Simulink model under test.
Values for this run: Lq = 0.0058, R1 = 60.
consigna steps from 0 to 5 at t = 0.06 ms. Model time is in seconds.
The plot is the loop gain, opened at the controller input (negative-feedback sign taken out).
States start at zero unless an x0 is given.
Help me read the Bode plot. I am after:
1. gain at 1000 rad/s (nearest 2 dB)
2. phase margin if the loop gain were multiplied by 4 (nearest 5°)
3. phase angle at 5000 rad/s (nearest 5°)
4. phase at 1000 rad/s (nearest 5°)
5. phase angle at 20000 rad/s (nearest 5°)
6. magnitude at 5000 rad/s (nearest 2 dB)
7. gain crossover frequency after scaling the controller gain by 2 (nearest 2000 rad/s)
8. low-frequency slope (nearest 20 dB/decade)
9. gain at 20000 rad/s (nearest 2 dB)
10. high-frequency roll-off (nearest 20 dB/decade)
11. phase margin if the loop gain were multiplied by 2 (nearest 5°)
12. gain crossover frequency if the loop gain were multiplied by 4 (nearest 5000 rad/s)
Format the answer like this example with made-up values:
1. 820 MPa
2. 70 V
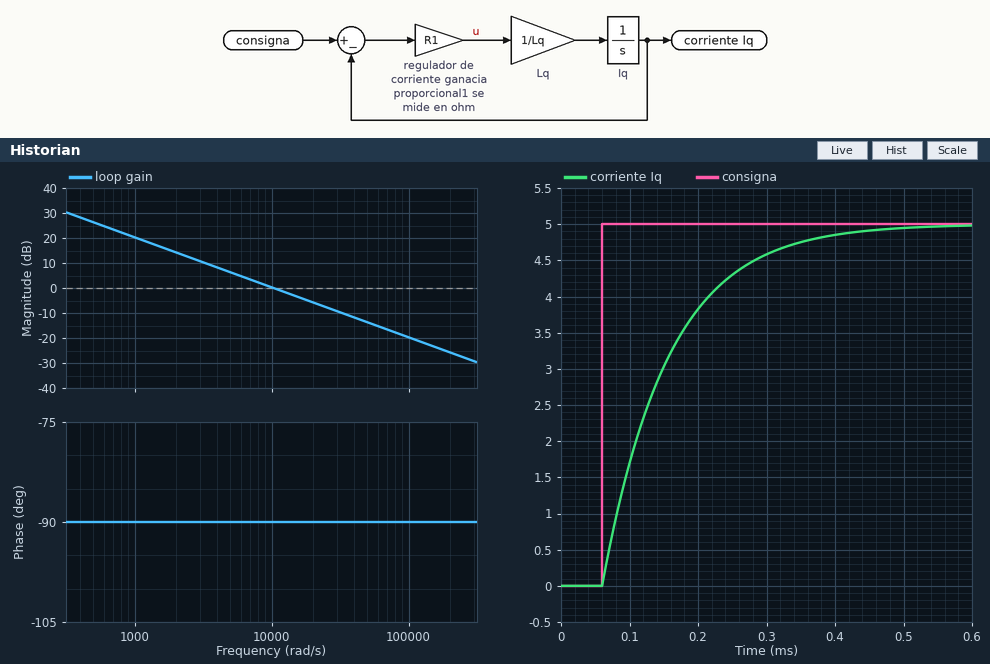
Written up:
1. 20 dB
2. 90°
3. -90°
4. -90°
5. -90°
6. 6 dB
7. 20000 rad/s
8. -20 dB/decade
9. -6 dB
10. -20 dB/decade
11. 90°
12. 40000 rad/s
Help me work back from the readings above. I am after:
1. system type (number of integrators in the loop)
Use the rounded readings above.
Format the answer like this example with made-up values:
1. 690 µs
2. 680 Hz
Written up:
1. 1
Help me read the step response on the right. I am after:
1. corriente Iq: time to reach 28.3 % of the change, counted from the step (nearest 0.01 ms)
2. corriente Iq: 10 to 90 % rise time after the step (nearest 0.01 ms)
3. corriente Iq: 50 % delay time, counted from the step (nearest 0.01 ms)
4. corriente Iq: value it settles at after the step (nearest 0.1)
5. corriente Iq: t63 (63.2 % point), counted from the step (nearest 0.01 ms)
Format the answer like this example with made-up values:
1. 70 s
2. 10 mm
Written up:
1. 0.03 ms
2. 0.21 ms
3. 0.07 ms
4. 5.0
5. 0.10 ms
